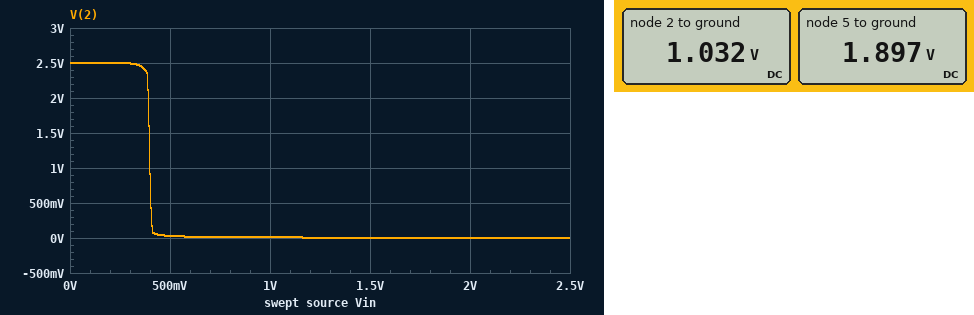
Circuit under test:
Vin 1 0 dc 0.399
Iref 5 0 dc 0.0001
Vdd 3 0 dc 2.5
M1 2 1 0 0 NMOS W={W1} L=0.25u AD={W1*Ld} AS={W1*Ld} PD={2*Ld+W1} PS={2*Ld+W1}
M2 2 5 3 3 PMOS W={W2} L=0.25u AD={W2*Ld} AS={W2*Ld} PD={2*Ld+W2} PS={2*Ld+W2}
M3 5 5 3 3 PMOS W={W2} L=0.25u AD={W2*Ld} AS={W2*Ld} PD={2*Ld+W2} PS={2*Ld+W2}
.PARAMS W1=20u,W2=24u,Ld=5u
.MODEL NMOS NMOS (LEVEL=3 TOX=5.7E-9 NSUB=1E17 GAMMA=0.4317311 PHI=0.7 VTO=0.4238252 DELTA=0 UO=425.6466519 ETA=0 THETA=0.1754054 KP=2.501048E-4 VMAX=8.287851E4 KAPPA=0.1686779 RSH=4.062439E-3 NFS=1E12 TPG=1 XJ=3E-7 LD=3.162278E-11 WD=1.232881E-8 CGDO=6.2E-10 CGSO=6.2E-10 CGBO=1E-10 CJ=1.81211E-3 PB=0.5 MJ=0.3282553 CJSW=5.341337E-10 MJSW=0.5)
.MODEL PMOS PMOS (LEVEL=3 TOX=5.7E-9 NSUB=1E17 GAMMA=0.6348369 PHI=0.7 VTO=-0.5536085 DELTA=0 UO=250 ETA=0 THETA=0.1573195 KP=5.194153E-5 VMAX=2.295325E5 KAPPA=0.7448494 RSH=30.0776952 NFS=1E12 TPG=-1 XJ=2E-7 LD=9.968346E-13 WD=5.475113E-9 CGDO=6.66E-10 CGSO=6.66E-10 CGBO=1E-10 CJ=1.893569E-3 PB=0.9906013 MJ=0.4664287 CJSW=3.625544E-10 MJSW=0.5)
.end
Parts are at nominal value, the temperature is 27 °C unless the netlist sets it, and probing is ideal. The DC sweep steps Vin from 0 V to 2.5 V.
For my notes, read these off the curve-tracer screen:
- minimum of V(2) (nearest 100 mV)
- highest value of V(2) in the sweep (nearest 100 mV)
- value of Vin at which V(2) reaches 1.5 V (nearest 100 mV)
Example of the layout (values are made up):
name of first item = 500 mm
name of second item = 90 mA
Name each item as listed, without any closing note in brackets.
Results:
minimum of V(2) = 0 V
highest value of V(2) in the sweep = 2.5 V
value of Vin at which V(2) reaches 1.5 V = 400 mV
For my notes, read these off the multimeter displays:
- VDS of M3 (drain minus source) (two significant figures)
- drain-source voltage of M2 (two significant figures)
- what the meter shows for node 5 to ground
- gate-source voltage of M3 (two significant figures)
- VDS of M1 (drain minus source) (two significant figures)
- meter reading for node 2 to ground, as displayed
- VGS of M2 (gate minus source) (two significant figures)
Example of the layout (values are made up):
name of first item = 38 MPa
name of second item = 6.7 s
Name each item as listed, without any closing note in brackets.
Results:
VDS of M3 (drain minus source) = -600 mV
drain-source voltage of M2 = -1.5 V
what the meter shows for node 5 to ground = 1.897 V
gate-source voltage of M3 = -600 mV
VDS of M1 (drain minus source) = 1.0 V
meter reading for node 2 to ground, as displayed = 1.032 V
VGS of M2 (gate minus source) = -600 mV
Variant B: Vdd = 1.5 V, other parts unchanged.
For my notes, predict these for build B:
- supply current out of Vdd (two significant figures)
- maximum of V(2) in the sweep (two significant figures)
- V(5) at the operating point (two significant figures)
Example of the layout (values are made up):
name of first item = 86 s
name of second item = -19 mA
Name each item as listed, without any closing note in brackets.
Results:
supply current out of Vdd = 200 µA
maximum of V(2) in the sweep = 1.5 V
V(5) at the operating point = 900 mV
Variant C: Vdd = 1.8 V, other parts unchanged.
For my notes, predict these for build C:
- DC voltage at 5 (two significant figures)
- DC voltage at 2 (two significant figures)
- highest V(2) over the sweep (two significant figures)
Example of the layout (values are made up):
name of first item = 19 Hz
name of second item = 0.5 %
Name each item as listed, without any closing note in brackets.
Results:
DC voltage at 5 = 1.2 V
DC voltage at 2 = 880 mV
highest V(2) over the sweep = 1.8 V
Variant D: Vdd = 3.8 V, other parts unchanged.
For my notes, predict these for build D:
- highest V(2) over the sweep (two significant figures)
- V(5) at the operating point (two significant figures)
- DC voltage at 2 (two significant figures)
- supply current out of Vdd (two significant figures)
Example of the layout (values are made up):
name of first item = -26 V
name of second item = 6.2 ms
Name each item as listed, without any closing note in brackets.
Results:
highest V(2) over the sweep = 3.8 V
V(5) at the operating point = 3.2 V
DC voltage at 2 = 1.3 V
supply current out of Vdd = 210 µA
